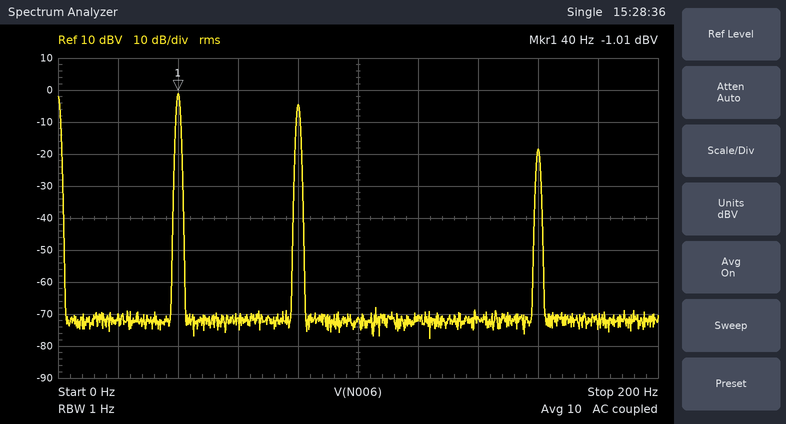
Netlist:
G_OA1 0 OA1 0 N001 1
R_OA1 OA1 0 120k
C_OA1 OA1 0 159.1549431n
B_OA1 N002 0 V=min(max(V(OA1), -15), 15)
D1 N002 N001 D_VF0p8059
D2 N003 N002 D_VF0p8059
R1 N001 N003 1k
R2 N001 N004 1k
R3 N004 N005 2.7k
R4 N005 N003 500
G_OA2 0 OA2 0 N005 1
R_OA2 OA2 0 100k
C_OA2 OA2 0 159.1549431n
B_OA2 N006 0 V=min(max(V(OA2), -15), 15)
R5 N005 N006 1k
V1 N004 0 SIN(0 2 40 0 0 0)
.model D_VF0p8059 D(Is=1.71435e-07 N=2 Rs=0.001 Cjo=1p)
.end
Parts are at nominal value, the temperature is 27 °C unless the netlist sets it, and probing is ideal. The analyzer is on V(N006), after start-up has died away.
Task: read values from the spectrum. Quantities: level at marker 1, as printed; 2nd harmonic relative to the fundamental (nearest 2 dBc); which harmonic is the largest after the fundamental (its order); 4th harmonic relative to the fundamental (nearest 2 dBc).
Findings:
-1.01 dBV
-4 dBc
2
-18 dBc
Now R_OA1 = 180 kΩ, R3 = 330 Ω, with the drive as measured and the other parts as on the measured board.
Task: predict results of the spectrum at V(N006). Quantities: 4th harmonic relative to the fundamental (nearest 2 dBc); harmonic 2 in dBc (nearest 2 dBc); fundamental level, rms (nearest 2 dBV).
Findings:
-28 dBc
-14 dBc
10 dBV
